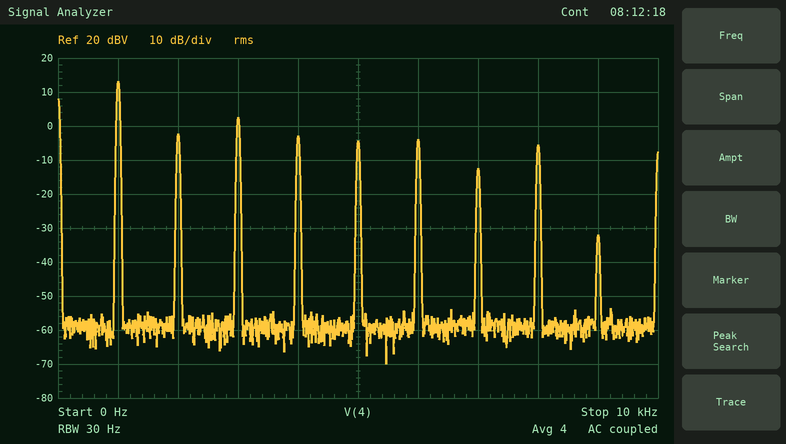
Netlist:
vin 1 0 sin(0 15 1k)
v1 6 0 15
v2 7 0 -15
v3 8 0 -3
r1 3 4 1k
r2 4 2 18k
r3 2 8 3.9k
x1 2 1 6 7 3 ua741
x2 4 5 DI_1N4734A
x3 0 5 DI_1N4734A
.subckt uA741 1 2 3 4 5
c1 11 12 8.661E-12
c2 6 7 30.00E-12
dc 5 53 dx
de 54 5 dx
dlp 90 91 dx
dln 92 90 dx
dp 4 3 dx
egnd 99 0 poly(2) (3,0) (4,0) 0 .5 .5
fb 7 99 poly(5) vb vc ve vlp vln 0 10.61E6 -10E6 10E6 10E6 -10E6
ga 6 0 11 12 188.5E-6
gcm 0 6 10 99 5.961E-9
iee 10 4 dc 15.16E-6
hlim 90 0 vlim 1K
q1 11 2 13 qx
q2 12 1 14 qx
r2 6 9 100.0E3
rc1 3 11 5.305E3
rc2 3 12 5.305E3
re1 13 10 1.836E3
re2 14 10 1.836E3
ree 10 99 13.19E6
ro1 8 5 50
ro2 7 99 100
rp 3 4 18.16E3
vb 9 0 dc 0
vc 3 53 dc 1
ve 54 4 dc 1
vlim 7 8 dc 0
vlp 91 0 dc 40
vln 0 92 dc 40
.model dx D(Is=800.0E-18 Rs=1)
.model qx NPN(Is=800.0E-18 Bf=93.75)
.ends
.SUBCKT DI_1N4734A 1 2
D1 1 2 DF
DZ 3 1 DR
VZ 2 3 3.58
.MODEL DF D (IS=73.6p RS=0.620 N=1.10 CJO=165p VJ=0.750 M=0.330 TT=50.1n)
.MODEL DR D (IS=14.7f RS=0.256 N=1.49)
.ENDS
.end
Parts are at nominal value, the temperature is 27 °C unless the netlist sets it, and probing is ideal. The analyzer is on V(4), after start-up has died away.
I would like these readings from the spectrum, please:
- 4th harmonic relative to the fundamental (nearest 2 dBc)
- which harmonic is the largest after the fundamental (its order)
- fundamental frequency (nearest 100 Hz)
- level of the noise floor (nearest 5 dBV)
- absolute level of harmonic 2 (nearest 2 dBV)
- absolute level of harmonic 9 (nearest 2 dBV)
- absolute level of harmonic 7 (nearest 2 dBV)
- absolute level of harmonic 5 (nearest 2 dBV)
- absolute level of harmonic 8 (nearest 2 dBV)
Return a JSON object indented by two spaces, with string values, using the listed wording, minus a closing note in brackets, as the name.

{
  "4th harmonic relative to the fundamental": "-16 dBc",
  "which harmonic is the largest after the fundamental": "3",
  "fundamental frequency": "1.0 kHz",
  "level of the noise floor": "-60 dBV",
  "absolute level of harmonic 2": "-2 dBV",
  "absolute level of harmonic 9": "-32 dBV",
  "absolute level of harmonic 7": "-12 dBV",
  "absolute level of harmonic 5": "-4 dBV",
  "absolute level of harmonic 8": "-6 dBV"
}
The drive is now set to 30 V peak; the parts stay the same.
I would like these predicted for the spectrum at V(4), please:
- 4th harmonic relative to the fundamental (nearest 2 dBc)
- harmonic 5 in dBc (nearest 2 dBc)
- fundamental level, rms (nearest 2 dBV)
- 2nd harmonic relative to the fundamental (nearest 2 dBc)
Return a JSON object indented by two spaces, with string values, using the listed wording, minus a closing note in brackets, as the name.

{
  "4th harmonic relative to the fundamental": "6 dBc",
  "harmonic 5 in dBc": "6 dBc",
  "fundamental level, rms": "-4 dBV",
  "2nd harmonic relative to the fundamental": "10 dBc"
}
